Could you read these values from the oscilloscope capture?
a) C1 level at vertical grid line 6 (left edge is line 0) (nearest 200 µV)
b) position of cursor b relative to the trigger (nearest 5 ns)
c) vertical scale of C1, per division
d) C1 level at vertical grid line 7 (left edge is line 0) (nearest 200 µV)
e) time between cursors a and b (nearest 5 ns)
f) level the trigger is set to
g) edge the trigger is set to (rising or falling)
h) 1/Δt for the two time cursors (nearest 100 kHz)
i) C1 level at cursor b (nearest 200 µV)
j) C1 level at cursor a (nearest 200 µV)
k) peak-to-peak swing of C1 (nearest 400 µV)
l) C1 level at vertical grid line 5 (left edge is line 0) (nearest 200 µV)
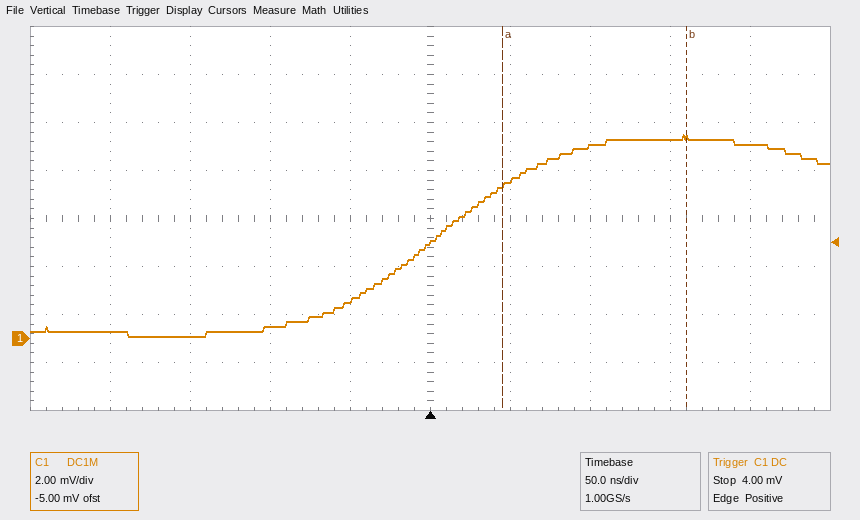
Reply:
6.6 mV
+160 ns
2 mV
8.0 mV
115 ns
4.00 mV
rising
8.7 MHz
8.4 mV
6.4 mV
8.4 mV
4.0 mV
